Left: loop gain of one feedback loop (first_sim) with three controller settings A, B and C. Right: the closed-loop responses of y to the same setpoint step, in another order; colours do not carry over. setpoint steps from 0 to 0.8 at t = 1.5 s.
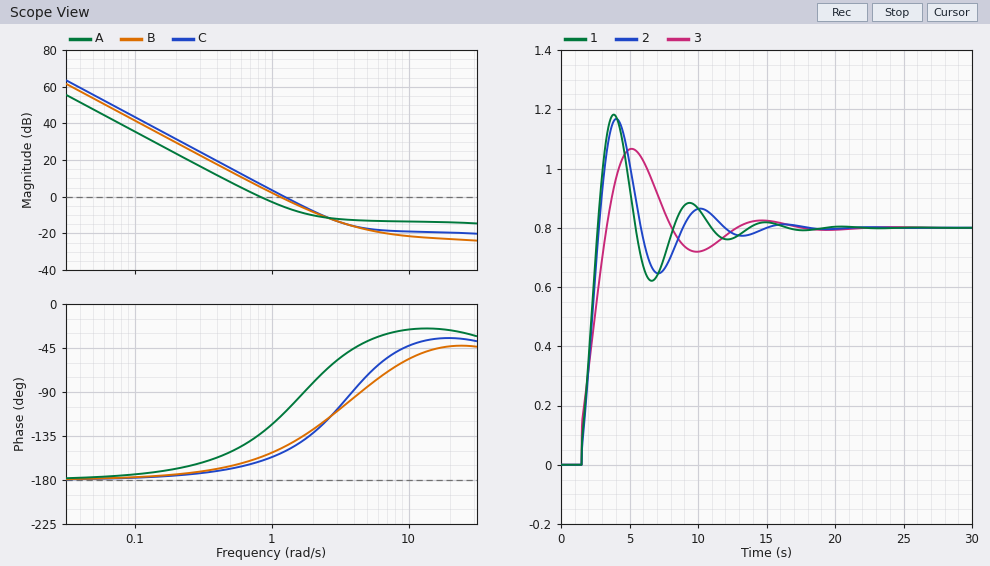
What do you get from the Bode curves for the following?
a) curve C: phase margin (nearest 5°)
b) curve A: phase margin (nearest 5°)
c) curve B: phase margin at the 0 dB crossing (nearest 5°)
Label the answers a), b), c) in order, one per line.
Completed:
a) 30°
b) 45°
c) 30°
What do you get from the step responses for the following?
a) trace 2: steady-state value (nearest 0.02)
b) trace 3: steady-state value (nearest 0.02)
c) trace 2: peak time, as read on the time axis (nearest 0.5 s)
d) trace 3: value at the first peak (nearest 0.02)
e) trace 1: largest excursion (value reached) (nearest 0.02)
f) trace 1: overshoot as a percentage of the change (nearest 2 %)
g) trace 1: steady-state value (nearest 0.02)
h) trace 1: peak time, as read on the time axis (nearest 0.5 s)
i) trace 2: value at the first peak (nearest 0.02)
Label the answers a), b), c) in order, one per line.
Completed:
a) 0.80
b) 0.80
c) 4.0 s
d) 1.06
e) 1.18
f) 48 %
g) 0.80
h) 4.0 s
i) 1.16
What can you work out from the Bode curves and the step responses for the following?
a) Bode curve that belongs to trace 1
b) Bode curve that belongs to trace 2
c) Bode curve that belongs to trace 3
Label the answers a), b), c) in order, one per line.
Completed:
a) C
b) B
c) A
